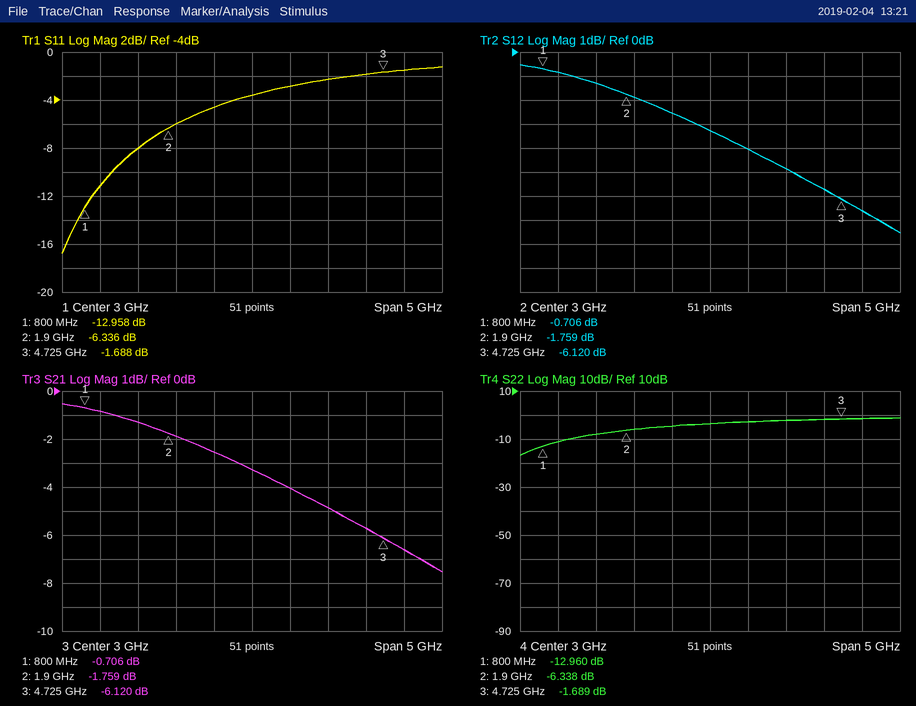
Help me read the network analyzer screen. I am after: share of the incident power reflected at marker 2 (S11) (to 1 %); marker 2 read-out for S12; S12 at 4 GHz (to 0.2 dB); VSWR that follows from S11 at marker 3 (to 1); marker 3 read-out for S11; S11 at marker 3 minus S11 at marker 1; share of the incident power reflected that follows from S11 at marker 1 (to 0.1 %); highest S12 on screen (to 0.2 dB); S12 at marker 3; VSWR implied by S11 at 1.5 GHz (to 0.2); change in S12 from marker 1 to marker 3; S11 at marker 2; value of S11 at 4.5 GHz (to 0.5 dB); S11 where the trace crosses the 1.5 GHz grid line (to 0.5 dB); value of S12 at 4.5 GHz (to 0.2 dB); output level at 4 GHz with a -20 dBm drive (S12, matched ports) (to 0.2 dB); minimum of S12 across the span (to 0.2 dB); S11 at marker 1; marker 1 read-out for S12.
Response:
23 %
-1.759 dB
-4.8 dB
10
-1.688 dB
11.270 dB
5.1 %
-0.6 dB
-6.120 dB
2.4
-5.414 dB
-6.336 dB
-2.0 dB
-8.0 dB
-5.8 dB
-24.8 dBm
-7.6 dB
-12.958 dB
-0.706 dB
